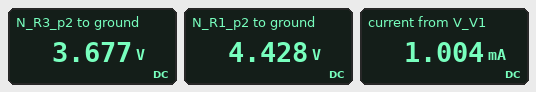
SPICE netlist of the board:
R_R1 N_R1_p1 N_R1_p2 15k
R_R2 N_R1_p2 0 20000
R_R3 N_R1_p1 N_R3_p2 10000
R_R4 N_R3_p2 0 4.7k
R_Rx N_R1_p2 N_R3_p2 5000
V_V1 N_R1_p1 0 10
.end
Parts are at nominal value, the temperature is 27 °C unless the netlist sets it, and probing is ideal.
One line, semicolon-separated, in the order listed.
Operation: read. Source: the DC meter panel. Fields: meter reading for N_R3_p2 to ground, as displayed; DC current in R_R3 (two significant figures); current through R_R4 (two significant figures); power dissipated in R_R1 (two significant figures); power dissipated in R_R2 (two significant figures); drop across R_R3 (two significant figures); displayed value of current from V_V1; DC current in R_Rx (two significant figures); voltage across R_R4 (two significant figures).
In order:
3.677 V; 630 µA; 780 µA; 2.1 mW; 980 µW; 6.3 V; 1.004 mA; 150 µA; 3.7 V
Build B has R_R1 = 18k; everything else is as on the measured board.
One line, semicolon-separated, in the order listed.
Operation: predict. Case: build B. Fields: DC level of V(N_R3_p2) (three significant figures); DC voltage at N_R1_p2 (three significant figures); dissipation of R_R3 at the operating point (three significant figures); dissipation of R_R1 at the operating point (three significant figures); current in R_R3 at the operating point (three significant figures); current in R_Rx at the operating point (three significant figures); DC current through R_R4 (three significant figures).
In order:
3.57 V; 4.16 V; 4.13 mW; 1.90 mW; 643 µA; 117 µA; 760 µA
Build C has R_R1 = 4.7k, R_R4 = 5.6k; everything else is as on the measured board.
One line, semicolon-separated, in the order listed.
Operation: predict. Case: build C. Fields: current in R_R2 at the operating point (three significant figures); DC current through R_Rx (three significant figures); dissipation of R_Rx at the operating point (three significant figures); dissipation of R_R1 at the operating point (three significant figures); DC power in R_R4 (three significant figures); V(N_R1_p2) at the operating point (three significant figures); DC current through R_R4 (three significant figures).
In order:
336 µA; 364 µA; 661 µW; 2.30 mW; 4.28 mW; 6.71 V; 874 µA
